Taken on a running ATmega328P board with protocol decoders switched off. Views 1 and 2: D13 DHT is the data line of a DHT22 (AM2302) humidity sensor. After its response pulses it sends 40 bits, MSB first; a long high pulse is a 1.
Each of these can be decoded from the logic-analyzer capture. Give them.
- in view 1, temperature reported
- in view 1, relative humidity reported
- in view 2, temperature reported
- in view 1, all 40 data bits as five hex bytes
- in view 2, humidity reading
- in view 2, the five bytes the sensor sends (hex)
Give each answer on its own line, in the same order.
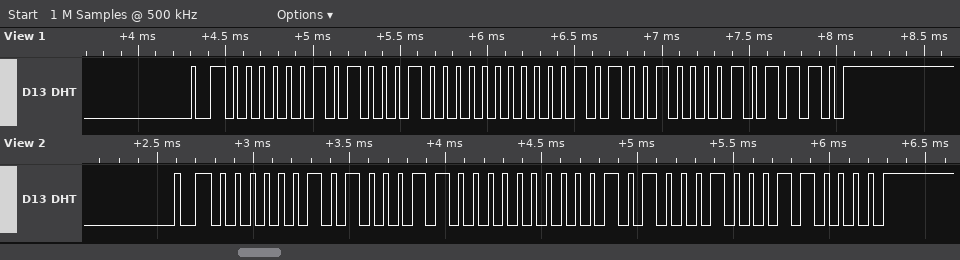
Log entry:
16.4 °C
64.8 %
16.2 °C
02 88 00 A4 2E
65.2 %
02 8C 00 A2 30
